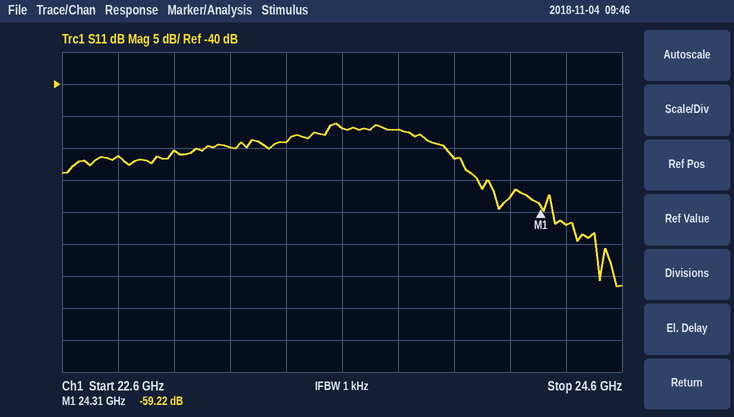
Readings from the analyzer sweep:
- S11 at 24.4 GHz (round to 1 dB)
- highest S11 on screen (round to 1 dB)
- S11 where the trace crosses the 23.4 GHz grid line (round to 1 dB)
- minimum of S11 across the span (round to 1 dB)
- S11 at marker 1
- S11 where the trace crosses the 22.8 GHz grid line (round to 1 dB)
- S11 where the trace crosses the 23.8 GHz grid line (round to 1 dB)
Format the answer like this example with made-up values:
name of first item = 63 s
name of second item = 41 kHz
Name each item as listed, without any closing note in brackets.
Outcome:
S11 at 24.4 GHz = -62 dB
highest S11 on screen = -46 dB
S11 where the trace crosses the 23.4 GHz grid line = -49 dB
minimum of S11 across the span = -72 dB
S11 at marker 1 = -59.22 dB
S11 where the trace crosses the 22.8 GHz grid line = -51 dB
S11 where the trace crosses the 23.8 GHz grid line = -47 dB
